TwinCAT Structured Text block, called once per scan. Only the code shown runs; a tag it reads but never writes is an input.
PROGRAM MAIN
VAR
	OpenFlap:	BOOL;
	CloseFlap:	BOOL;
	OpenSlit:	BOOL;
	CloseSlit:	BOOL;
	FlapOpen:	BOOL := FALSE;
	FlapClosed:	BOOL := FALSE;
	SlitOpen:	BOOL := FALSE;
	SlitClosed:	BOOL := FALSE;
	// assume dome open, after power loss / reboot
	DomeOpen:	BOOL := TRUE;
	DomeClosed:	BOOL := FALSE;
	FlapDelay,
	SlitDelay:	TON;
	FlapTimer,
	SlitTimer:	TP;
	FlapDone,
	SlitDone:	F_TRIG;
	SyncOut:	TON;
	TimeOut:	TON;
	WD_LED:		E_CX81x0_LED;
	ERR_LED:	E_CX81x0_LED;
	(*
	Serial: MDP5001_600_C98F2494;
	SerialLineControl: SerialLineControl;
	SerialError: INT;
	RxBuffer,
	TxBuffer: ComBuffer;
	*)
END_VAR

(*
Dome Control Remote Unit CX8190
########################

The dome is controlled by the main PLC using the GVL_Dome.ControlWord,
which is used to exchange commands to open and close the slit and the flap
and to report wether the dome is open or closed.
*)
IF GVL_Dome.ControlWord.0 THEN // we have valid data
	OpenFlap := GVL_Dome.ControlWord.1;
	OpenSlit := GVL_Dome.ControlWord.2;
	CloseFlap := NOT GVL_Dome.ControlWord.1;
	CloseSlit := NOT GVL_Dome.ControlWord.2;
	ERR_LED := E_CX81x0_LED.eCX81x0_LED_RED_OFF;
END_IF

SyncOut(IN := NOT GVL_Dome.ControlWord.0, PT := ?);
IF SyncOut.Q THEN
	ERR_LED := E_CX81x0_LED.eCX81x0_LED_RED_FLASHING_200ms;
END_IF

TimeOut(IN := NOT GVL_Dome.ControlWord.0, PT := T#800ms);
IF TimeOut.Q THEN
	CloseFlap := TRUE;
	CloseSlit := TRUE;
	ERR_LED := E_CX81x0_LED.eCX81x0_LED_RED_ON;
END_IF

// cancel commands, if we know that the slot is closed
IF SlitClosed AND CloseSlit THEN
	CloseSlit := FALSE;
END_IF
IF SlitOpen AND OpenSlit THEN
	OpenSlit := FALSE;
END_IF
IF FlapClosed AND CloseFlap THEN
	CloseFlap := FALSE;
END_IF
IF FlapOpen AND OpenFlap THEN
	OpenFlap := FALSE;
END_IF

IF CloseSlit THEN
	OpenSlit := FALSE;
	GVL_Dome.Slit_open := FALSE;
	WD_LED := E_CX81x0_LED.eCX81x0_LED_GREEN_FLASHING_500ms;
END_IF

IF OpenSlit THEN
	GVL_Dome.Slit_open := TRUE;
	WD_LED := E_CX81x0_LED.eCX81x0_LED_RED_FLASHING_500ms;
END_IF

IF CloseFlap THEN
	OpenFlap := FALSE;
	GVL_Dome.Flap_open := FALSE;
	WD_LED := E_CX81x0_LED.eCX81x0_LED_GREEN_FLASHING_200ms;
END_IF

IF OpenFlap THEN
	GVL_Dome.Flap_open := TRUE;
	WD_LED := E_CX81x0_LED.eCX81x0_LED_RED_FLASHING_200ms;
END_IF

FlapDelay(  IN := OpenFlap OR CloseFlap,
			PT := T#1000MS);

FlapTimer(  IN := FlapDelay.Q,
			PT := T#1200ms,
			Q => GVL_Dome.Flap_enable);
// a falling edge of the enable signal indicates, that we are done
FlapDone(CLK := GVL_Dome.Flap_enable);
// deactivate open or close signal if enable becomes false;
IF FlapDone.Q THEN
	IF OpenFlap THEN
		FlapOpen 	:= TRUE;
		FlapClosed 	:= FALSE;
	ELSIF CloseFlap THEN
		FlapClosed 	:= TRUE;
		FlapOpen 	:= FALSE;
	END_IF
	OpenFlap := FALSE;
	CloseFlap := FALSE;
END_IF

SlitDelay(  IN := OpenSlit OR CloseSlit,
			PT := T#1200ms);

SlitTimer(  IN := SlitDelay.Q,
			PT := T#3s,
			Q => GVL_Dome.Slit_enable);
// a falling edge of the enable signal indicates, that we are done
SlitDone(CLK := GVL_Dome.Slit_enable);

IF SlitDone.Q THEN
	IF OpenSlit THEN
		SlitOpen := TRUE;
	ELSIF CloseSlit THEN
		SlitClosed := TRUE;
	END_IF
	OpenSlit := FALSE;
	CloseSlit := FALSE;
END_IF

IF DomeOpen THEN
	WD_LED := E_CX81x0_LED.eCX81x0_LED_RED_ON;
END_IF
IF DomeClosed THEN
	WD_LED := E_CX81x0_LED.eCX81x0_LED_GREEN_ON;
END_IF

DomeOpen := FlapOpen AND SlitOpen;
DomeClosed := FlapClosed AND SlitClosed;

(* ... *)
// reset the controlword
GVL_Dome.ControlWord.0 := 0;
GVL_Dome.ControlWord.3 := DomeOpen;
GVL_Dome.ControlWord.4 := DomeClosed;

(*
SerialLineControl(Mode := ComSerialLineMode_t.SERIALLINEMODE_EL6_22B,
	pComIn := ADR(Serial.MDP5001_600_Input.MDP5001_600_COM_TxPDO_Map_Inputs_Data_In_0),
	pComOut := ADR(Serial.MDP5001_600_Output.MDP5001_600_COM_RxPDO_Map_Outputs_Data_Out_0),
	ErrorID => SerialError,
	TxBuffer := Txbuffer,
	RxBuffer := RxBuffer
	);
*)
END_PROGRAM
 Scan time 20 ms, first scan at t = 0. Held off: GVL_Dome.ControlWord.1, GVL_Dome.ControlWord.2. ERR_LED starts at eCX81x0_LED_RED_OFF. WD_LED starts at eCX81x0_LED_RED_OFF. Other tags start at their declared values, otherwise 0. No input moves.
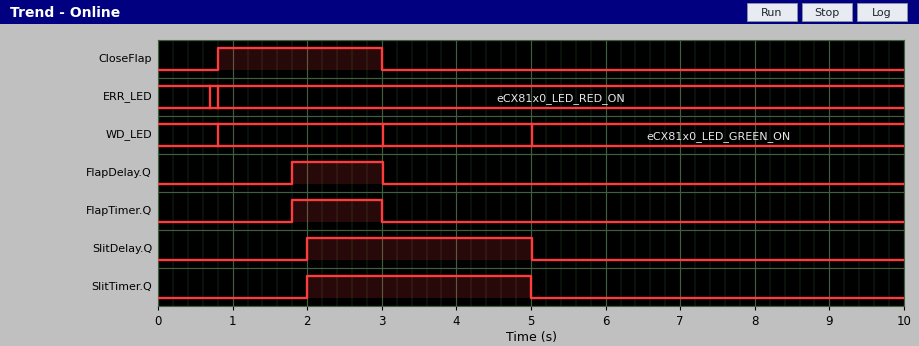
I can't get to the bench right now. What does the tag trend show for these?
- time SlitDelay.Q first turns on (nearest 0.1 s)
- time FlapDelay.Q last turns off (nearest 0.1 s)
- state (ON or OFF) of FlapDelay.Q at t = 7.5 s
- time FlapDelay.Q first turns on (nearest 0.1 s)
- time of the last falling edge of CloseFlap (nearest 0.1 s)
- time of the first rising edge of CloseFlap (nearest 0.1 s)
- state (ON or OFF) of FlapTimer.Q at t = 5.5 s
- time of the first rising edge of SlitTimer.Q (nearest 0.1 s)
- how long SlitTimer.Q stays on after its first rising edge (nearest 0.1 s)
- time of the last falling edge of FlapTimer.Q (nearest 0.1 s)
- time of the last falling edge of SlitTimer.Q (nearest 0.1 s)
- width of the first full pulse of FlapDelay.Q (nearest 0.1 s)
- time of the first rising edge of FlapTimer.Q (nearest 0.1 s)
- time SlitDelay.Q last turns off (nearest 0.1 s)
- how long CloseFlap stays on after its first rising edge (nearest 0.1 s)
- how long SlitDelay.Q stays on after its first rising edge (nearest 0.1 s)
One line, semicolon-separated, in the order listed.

2.0 s; 3.0 s; OFF; 1.8 s; 3.0 s; 0.8 s; OFF; 2.0 s; 3.0 s; 3.0 s; 5.0 s; 1.2 s; 1.8 s; 5.0 s; 2.2 s; 3.0 s
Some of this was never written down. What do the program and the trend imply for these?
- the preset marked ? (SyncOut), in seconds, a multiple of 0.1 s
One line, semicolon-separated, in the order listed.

0.7 s
